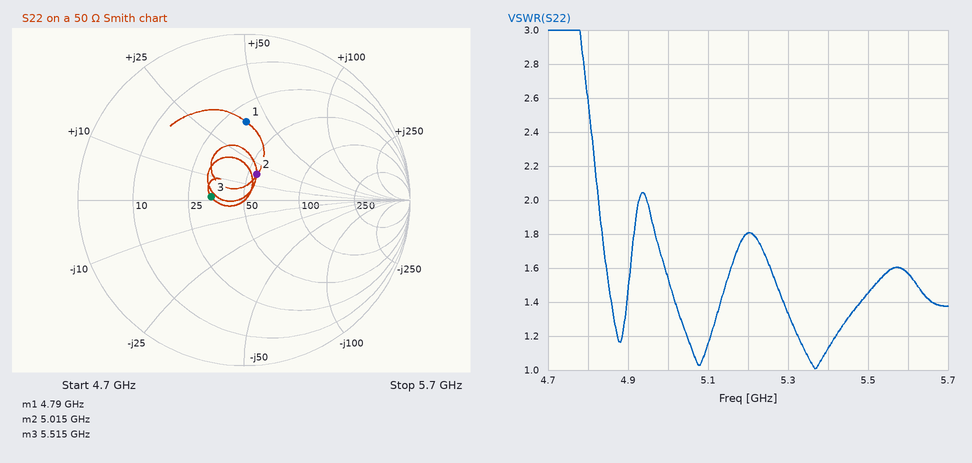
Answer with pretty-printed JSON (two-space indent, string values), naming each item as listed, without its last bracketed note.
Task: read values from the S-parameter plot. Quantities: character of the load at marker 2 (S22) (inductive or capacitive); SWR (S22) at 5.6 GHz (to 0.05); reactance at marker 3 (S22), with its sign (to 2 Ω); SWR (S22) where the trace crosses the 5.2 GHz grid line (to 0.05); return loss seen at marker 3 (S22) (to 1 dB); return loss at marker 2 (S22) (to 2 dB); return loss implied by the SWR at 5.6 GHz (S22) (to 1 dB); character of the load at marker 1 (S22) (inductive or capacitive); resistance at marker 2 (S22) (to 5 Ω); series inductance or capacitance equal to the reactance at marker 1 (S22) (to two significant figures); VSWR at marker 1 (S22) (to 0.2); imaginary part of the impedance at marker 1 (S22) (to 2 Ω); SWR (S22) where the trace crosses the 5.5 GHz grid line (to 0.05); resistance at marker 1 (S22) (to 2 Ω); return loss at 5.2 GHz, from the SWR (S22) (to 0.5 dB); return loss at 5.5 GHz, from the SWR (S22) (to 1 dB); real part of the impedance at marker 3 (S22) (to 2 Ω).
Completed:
{
  "character of the load at marker 2 (S22)": "inductive",
  "SWR (S22) at 5.6 GHz": "1.55",
  "reactance at marker 3 (S22), with its sign": "+2 Ω",
  "SWR (S22) where the trace crosses the 5.2 GHz grid line": "1.80",
  "return loss seen at marker 3 (S22)": "14 dB",
  "return loss at marker 2 (S22)": "16 dB",
  "return loss implied by the SWR at 5.6 GHz (S22)": "13 dB",
  "character of the load at marker 1 (S22)": "inductive",
  "resistance at marker 2 (S22)": "55 Ω",
  "series inductance or capacitance equal to the reactance at marker 1 (S22)": "1.3 nH",
  "VSWR at marker 1 (S22)": "2.8",
  "imaginary part of the impedance at marker 1 (S22)": "+40 Ω",
  "SWR (S22) where the trace crosses the 5.5 GHz grid line": "1.45",
  "resistance at marker 1 (S22)": "32 Ω",
  "return loss at 5.2 GHz, from the SWR (S22)": "11.0 dB",
  "return loss at 5.5 GHz, from the SWR (S22)": "15 dB",
  "real part of the impedance at marker 3 (S22)": "34 Ω"
}
